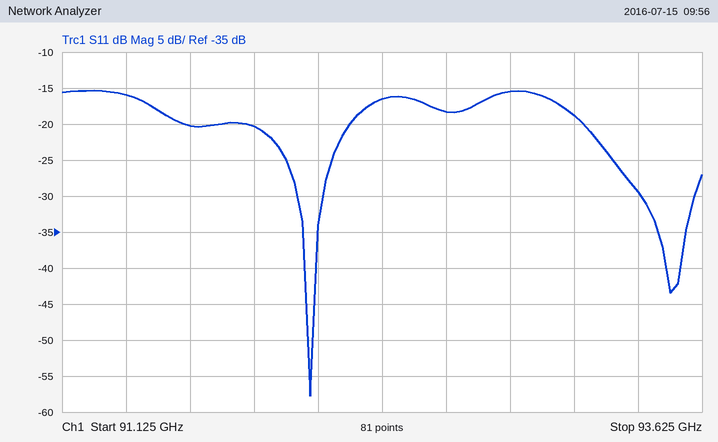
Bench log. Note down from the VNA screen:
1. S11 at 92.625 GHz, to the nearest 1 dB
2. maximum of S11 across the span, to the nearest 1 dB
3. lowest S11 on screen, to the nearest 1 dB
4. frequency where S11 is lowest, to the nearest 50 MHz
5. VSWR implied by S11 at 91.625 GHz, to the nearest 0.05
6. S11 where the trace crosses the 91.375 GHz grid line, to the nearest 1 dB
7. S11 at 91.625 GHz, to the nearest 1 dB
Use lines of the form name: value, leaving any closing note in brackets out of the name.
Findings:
S11 at 92.625 GHz, to the nearest 1 dB: -18 dB
maximum of S11 across the span, to the nearest 1 dB: -15 dB
lowest S11 on screen, to the nearest 1 dB: -58 dB
frequency where S11 is lowest, to the nearest 50 MHz: 92.10 GHz
VSWR implied by S11 at 91.625 GHz, to the nearest 0.05: 1.20
S11 where the trace crosses the 91.375 GHz grid line, to the nearest 1 dB: -16 dB
S11 at 91.625 GHz, to the nearest 1 dB: -20 dB
